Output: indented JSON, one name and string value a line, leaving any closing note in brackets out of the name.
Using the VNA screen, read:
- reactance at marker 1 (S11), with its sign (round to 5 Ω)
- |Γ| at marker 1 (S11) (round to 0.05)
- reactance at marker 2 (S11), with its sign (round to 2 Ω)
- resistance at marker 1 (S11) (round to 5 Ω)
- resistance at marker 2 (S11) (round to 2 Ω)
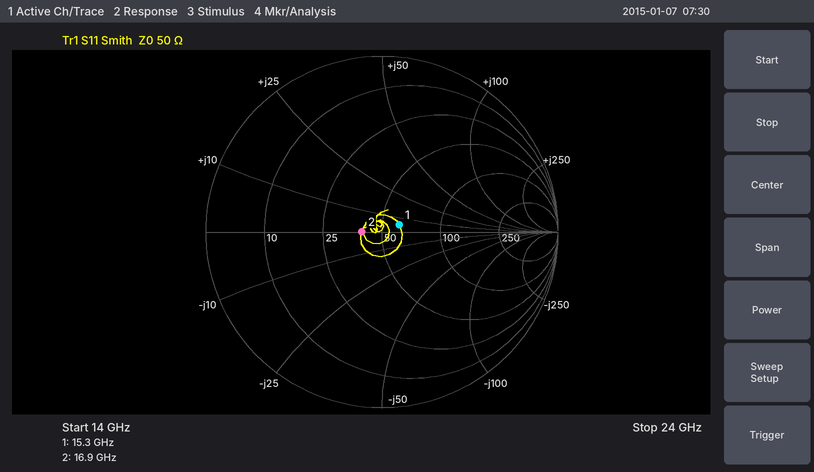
{
  "reactance at marker 1 (S11), with its sign": "+5 Ω",
  "|Γ| at marker 1 (S11)": "0.10",
  "reactance at marker 2 (S11), with its sign": "0 Ω",
  "resistance at marker 1 (S11)": "60 Ω",
  "resistance at marker 2 (S11)": "40 Ω"
}
